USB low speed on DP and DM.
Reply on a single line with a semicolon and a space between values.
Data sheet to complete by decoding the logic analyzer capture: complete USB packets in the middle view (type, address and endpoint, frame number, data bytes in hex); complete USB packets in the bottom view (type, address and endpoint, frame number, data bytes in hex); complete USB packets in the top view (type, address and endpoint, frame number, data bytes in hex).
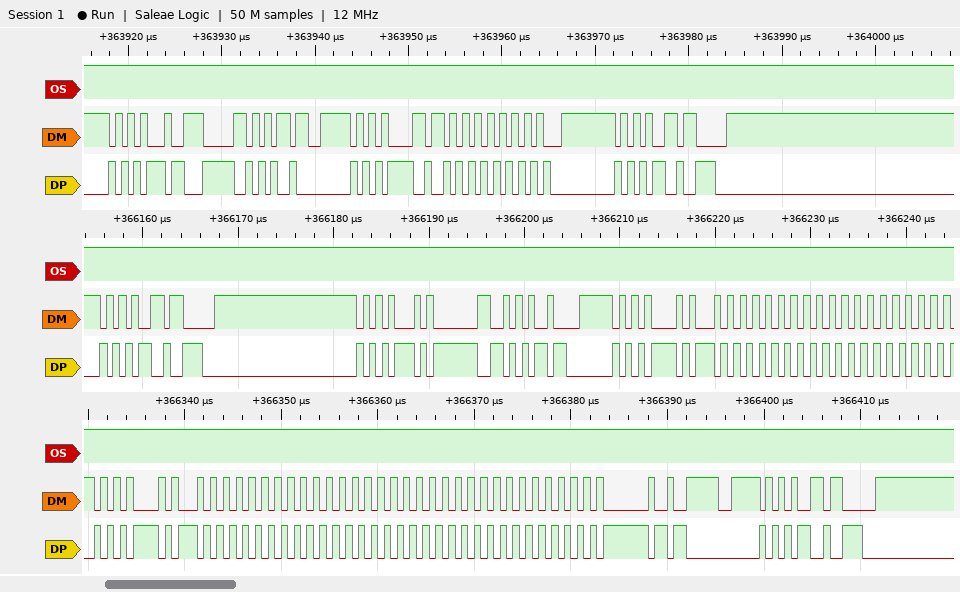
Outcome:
ACK, OUT ADDR 47 EP 0; DATA0 [ 00 00 00 00 00 00 00 00 ], ACK; IN ADDR 47 EP 0, DATA1 [ ], ACK
